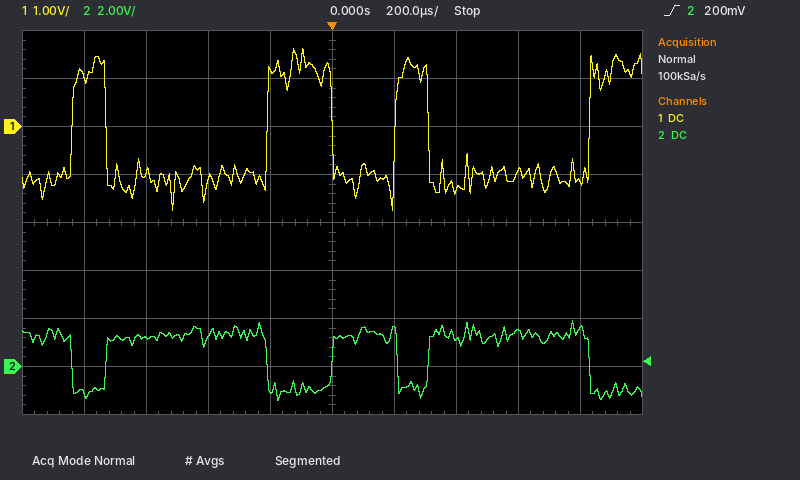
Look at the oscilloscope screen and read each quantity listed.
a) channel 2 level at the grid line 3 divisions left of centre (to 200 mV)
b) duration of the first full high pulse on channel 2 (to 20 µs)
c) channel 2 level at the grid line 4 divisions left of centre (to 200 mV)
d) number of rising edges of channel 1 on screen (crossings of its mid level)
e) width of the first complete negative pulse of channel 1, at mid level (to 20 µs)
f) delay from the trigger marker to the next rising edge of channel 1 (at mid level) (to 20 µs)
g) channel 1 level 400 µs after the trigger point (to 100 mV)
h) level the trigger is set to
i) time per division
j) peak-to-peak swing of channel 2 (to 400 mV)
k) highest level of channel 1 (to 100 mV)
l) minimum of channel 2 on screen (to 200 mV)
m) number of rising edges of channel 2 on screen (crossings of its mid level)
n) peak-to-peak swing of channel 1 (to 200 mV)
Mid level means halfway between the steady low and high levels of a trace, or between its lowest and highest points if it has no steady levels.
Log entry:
1.2 V
520 µs
-1.2 V
4
520 µs
200 µs
-1.3 V
200 mV
200 µs
3.2 V
1.6 V
-1.4 V
3
3.4 V
